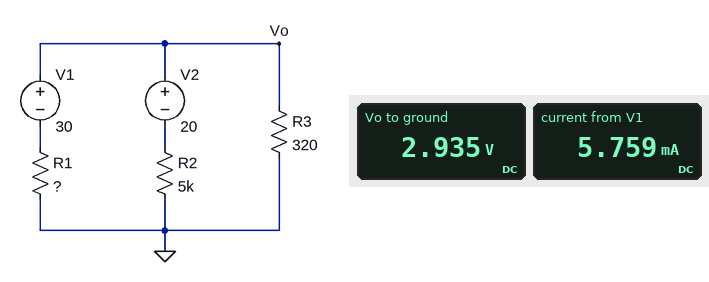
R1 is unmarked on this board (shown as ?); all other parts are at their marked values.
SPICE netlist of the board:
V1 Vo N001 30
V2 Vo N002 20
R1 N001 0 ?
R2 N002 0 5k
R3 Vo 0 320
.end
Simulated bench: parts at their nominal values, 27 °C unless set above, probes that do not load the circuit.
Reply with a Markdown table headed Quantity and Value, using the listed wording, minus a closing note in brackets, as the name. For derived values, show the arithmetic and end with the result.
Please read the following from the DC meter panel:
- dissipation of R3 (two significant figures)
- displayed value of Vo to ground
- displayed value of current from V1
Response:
| Quantity | Value |
|---|---|
| dissipation of R3 | (2.935 V)^2 / 320 Ω = 27 mW |
| displayed value of Vo to ground | 2.935 V |
| displayed value of current from V1 | 5.759 mA |
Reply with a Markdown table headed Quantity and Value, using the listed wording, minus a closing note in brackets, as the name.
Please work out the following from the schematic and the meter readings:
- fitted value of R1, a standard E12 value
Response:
| Quantity | Value |
|---|---|
| fitted value of R1, a standard E12 value | 4.7 kΩ |
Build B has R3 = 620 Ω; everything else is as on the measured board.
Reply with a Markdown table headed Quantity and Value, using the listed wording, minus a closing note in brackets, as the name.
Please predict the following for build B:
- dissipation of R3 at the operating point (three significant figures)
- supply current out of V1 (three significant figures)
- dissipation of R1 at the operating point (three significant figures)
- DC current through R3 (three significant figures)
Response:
| Quantity | Value |
|---|---|
| dissipation of R3 at the operating point | 42.4 mW |
| supply current out of V1 | 5.29 mA |
| dissipation of R1 at the operating point | 132 mW |
| DC current through R3 | 8.27 mA |
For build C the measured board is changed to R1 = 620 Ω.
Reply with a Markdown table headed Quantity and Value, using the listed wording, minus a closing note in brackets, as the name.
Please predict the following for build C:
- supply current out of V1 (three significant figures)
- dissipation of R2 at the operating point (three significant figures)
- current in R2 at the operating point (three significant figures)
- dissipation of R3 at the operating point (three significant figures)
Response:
| Quantity | Value |
|---|---|
| supply current out of V1 | 31.3 mA |
| dissipation of R2 at the operating point | 17.6 mW |
| current in R2 at the operating point | 1.88 mA |
| dissipation of R3 at the operating point | 352 mW |
